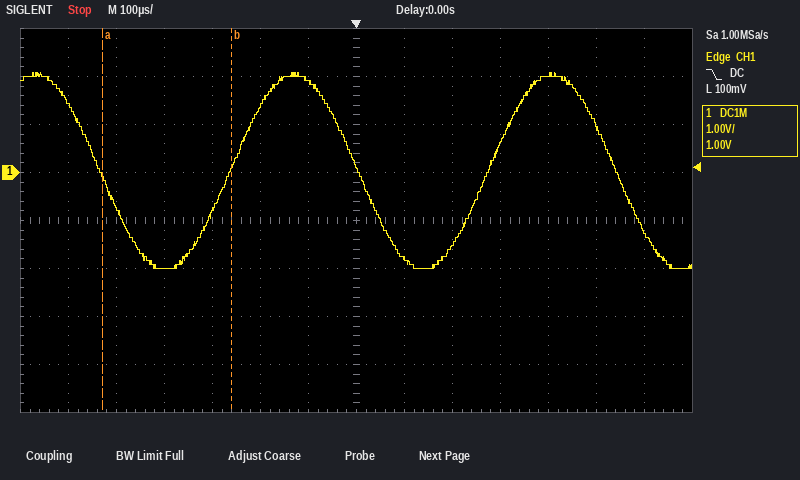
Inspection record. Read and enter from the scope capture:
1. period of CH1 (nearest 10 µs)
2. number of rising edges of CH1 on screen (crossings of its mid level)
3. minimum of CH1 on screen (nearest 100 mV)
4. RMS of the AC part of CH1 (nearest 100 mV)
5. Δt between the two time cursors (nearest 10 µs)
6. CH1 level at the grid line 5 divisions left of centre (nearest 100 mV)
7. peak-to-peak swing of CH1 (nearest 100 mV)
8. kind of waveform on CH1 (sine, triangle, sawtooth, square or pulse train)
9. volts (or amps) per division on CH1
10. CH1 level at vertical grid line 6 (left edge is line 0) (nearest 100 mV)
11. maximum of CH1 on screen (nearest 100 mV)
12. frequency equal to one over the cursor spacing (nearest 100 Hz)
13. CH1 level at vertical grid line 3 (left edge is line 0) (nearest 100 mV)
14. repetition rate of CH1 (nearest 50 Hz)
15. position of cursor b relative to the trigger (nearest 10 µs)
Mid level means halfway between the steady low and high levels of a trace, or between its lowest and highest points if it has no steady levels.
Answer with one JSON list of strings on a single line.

["540 µs", "2", "-2.0 V", "1.4 V", "270 µs", "-700 mV", "4.1 V", "sine", "1 V", "1.9 V", "2.1 V", "3.7 kHz", "-2.0 V", "1.85 kHz", "-260 µs"]
